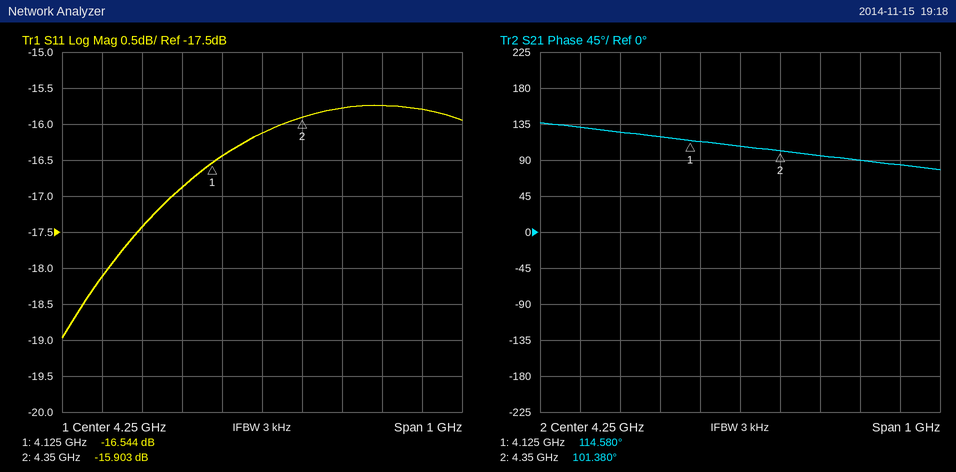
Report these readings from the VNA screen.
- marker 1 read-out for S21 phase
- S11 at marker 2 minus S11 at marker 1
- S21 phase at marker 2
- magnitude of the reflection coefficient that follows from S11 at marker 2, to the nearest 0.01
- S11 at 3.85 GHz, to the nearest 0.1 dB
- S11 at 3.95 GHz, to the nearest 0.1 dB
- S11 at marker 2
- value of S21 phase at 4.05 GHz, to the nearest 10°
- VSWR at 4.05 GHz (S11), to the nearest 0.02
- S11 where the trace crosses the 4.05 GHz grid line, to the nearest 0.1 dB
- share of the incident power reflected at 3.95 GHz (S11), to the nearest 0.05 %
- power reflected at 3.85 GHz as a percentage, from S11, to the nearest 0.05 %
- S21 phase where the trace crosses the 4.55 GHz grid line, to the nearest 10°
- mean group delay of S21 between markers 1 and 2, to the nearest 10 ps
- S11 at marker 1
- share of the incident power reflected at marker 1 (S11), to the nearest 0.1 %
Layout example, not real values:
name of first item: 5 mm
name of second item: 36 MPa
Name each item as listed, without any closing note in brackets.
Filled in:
marker 1 read-out for S21 phase: 114.580°
S11 at marker 2 minus S11 at marker 1: 0.641 dB
S21 phase at marker 2: 101.380°
magnitude of the reflection coefficient that follows from S11 at marker 2, to the nearest 0.01: 0.16
S11 at 3.85 GHz, to the nearest 0.1 dB: -18.1 dB
S11 at 3.95 GHz, to the nearest 0.1 dB: -17.4 dB
S11 at marker 2: -15.903 dB
value of S21 phase at 4.05 GHz, to the nearest 10°: 120°
VSWR at 4.05 GHz (S11), to the nearest 0.02: 1.34
S11 where the trace crosses the 4.05 GHz grid line, to the nearest 0.1 dB: -16.9 dB
share of the incident power reflected at 3.95 GHz (S11), to the nearest 0.05 %: 1.80 %
power reflected at 3.85 GHz as a percentage, from S11, to the nearest 0.05 %: 1.55 %
S21 phase where the trace crosses the 4.55 GHz grid line, to the nearest 10°: 90°
mean group delay of S21 between markers 1 and 2, to the nearest 10 ps: 160 ps
S11 at marker 1: -16.544 dB
share of the incident power reflected at marker 1 (S11), to the nearest 0.1 %: 2.2 %
